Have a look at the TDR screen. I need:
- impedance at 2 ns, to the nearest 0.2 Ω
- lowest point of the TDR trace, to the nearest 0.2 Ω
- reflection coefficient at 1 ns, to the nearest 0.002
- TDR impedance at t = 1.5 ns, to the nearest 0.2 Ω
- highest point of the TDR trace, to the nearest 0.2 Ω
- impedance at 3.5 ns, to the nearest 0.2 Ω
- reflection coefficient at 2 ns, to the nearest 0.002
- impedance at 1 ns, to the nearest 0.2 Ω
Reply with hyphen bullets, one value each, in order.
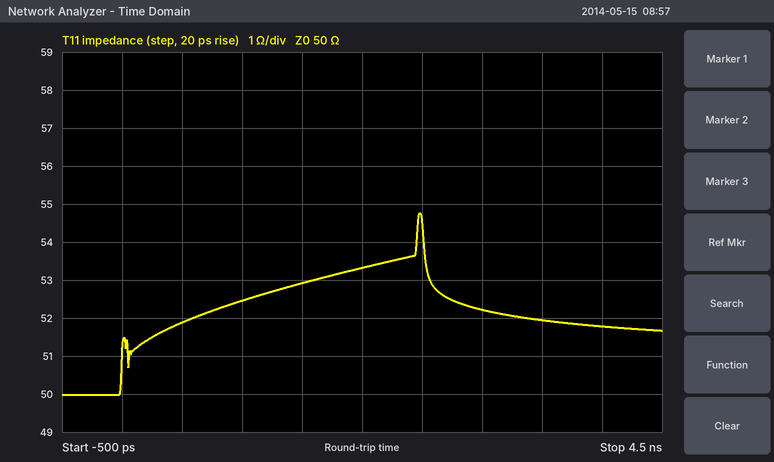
- 53.4 Ω
- 50.0 Ω
- +0.024
- 53.0 Ω
- 54.8 Ω
- 52.0 Ω
- +0.032
- 52.4 Ω
